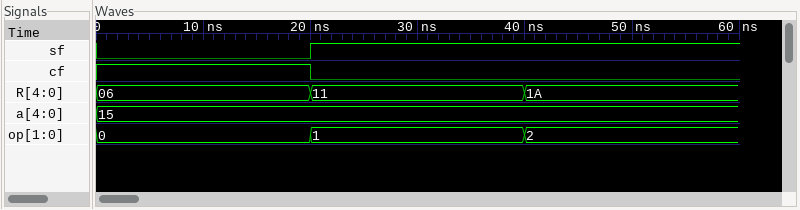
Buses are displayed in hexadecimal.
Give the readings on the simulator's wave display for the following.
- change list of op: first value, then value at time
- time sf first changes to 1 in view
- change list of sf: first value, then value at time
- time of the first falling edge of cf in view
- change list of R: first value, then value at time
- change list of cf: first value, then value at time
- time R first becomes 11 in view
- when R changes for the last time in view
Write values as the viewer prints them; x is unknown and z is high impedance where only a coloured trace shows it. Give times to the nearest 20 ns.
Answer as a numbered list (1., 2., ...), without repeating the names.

1. 0, 1 at 20 ns, 2 at 40 ns
2. 20 ns
3. 0, 1 at 20 ns
4. 20 ns
5. 06, 11 at 20 ns, 1A at 40 ns
6. 1, 0 at 20 ns
7. 20 ns
8. 40 ns
